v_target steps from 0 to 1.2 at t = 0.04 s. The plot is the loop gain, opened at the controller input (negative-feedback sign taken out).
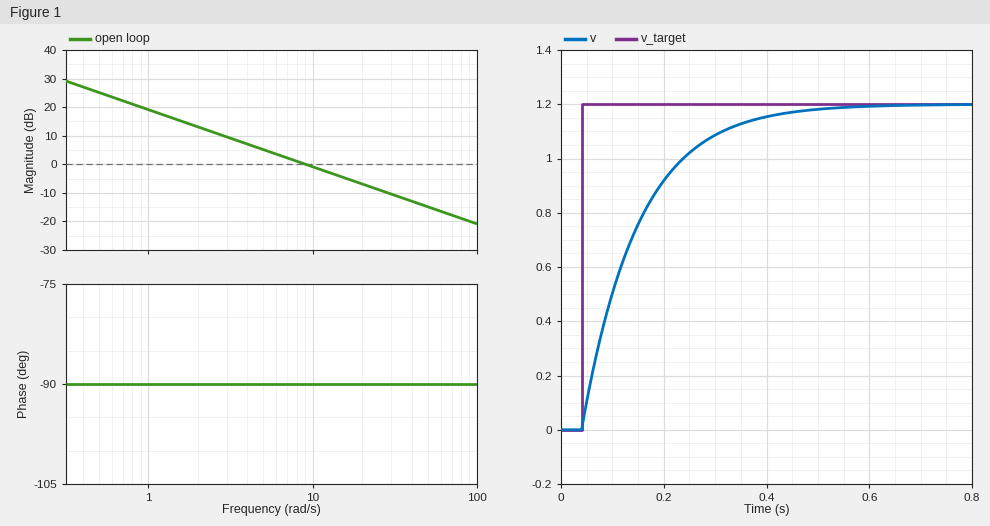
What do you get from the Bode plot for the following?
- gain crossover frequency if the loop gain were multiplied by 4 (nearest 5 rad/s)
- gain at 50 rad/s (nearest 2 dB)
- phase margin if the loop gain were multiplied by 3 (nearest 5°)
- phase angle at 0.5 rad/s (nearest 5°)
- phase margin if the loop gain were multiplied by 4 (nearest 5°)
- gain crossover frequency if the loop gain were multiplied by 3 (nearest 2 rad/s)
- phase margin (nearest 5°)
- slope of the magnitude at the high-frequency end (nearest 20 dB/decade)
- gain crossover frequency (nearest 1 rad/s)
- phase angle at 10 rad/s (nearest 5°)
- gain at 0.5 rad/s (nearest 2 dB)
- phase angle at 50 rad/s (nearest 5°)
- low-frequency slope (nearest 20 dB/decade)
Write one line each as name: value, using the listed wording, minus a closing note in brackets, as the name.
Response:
gain crossover frequency if the loop gain were multiplied by 4: 35 rad/s
gain at 50 rad/s: -14 dB
phase margin if the loop gain were multiplied by 3: 90°
phase angle at 0.5 rad/s: -90°
phase margin if the loop gain were multiplied by 4: 90°
gain crossover frequency if the loop gain were multiplied by 3: 28 rad/s
phase margin: 90°
slope of the magnitude at the high-frequency end: -20 dB/decade
gain crossover frequency: 9 rad/s
phase angle at 10 rad/s: -90°
gain at 0.5 rad/s: 26 dB
phase angle at 50 rad/s: -90°
low-frequency slope: -20 dB/decade
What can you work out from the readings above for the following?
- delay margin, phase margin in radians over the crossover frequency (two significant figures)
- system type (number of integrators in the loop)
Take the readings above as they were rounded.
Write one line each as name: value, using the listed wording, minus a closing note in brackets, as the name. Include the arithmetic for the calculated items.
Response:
delay margin, phase margin in radians over the crossover frequency: 90 × π / 180 / 9 = 0.17 s
system type: 1
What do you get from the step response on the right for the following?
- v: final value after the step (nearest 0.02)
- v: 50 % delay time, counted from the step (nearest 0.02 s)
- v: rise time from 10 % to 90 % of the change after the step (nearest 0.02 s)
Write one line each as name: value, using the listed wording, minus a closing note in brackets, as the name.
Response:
v: final value after the step: 1.20
v: 50 % delay time, counted from the step: 0.08 s
v: rise time from 10 % to 90 % of the change after the step: 0.24 s
